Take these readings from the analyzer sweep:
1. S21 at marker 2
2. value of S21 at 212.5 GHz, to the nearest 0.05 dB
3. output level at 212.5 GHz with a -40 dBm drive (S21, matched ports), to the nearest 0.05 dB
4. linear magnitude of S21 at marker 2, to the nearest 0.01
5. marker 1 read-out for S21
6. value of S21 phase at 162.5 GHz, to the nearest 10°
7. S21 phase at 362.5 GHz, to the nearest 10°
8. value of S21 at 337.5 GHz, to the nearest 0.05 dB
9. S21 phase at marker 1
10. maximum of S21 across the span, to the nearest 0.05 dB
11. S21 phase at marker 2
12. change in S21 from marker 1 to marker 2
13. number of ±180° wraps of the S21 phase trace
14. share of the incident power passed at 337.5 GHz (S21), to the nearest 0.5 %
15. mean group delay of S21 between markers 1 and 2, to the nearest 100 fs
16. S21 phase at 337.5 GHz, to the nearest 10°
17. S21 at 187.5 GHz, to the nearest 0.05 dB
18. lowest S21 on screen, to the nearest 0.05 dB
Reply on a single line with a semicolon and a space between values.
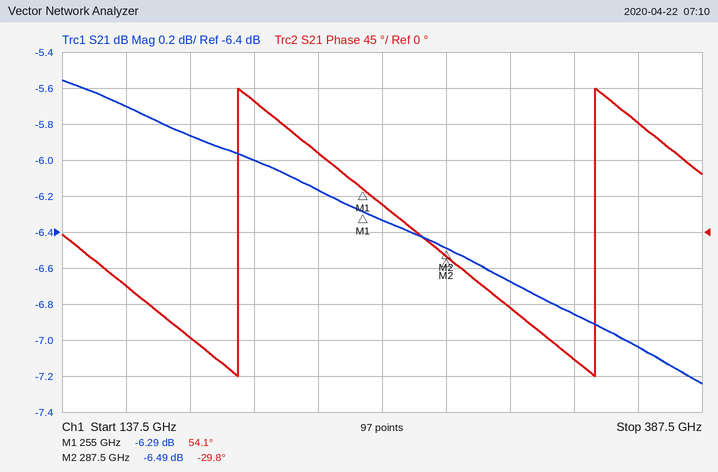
-6.49 dB; -6.00 dB; -46.00 dBm; 0.47; -6.29 dB; -70°; 140°; -6.85 dB; 54.1°; -5.55 dB; -29.8°; -0.20 dB; 2; 20.5 %; 7.2 ps; -160°; -5.85 dB; -7.25 dB
